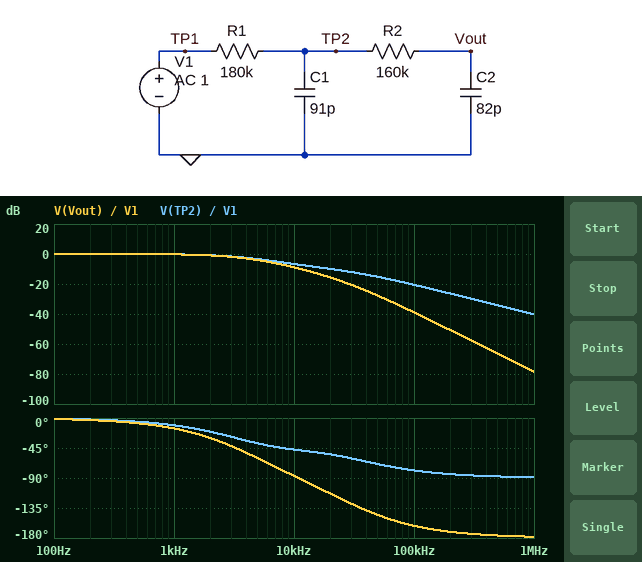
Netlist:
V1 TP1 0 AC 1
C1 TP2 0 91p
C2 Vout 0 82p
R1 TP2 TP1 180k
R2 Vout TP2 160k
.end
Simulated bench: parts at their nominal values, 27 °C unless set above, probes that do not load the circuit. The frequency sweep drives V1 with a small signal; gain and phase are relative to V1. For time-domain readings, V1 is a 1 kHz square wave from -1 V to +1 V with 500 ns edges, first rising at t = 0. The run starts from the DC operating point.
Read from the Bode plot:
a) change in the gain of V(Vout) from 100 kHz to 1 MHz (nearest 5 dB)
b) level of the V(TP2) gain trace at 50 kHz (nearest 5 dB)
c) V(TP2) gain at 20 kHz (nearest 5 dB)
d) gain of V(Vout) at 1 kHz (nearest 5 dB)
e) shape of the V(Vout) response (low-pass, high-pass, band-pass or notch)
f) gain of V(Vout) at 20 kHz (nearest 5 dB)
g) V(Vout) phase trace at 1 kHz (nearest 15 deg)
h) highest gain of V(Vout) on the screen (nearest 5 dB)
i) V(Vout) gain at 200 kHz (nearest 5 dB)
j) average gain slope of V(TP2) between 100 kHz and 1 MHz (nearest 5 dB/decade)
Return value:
-40 dB
-15 dB
-10 dB
0 dB
low-pass
-15 dB
-15 deg
0 dB
-50 dB
-20 dB/decade
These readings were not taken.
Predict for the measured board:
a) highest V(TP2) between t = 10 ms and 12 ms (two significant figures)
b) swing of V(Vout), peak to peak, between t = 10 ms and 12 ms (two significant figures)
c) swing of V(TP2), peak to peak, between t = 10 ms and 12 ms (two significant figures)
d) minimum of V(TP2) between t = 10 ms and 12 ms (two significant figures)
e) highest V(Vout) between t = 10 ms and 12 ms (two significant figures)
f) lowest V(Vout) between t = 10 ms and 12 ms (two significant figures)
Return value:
1.0 V
2.0 V
2.0 V
-1.0 V
1.0 V
-1.0 V
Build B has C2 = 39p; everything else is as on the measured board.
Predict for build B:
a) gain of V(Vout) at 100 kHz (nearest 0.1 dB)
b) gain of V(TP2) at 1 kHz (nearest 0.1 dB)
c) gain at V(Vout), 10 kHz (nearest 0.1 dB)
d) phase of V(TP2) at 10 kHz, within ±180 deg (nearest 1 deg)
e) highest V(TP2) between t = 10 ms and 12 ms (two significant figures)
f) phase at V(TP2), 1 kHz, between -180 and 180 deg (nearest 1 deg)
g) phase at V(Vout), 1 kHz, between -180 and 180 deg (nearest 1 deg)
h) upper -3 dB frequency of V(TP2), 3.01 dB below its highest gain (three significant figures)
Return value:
-32.8 dB
-0.1 dB
-5.8 dB
-51 deg
1.0 V
-8 deg
-11 deg
6.43 kHz
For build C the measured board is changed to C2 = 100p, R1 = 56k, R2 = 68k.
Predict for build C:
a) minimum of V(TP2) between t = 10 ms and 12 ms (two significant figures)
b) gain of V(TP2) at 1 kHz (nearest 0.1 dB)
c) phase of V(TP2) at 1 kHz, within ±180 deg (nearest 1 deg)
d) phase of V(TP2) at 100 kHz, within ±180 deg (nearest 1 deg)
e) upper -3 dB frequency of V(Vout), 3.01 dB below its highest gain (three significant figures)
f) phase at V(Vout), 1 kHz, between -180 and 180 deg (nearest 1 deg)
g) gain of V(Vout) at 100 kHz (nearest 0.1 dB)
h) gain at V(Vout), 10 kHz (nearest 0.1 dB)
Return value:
-1.0 V
0 dB
-4 deg
-62 deg
10.2 kHz
-6 deg
-24.5 dB
-2.9 dB
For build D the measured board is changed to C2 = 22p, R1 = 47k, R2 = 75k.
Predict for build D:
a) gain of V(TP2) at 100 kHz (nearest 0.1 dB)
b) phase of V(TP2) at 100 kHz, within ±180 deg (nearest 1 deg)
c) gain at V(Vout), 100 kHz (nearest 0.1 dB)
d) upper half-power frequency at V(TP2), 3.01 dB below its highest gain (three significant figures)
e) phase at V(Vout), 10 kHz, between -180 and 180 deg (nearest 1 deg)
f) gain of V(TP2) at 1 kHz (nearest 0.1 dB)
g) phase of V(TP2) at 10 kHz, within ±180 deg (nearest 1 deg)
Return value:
-10.3 dB
-66 deg
-13.5 dB
28.8 kHz
-24 deg
0 dB
-18 deg
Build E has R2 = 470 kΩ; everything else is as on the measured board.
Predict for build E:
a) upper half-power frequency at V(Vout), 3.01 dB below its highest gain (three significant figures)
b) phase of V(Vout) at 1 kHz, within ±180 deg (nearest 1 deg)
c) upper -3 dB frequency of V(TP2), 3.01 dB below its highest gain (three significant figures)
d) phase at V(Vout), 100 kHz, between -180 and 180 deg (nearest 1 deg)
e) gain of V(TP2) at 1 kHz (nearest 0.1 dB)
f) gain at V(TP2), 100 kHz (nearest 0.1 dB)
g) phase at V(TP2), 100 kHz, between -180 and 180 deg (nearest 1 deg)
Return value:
2.62 kHz
-24 deg
5.00 kHz
-170 deg
-0.3 dB
-20.3 dB
-82 deg
